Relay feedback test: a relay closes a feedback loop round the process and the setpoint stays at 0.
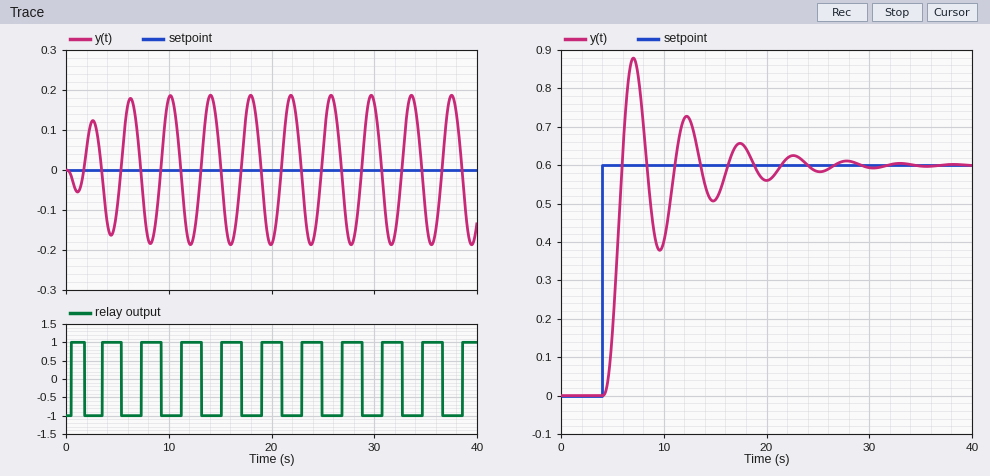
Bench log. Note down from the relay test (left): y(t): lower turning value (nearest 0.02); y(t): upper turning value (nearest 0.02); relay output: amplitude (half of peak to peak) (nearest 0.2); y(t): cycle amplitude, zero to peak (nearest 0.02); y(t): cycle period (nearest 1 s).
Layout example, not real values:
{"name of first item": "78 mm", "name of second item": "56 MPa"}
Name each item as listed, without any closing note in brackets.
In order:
{"y(t): lower turning value": "-0.18", "y(t): upper turning value": "0.18", "relay output: amplitude (half of peak to peak)": "1.0", "y(t): cycle amplitude, zero to peak": "0.18", "y(t): cycle period": "4 s"}
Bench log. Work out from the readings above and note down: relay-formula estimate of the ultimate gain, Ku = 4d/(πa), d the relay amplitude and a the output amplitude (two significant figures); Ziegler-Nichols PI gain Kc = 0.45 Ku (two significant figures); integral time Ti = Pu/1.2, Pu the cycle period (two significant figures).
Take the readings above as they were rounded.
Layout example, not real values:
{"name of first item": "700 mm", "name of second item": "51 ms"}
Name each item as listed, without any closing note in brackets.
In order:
{"relay-formula estimate of the ultimate gain, Ku = 4d/(πa), d the relay amplitude and a the output amplitude": "7.1", "Ziegler-Nichols PI gain Kc = 0.45 Ku": "3.2", "integral time Ti = Pu/1.2, Pu the cycle period": "3.3 s"}
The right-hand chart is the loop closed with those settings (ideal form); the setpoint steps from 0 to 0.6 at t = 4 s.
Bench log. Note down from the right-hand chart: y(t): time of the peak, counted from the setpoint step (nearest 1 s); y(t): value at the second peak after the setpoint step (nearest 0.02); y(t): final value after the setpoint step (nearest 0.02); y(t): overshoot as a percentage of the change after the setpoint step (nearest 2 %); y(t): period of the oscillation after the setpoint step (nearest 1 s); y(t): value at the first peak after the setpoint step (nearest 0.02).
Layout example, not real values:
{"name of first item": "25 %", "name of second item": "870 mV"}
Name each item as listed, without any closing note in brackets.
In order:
{"y(t): time of the peak, counted from the setpoint step": "3 s", "y(t): value at the second peak after the setpoint step": "0.72", "y(t): final value after the setpoint step": "0.60", "y(t): overshoot as a percentage of the change after the setpoint step": "46 %", "y(t): period of the oscillation after the setpoint step": "5 s", "y(t): value at the first peak after the setpoint step": "0.88"}
